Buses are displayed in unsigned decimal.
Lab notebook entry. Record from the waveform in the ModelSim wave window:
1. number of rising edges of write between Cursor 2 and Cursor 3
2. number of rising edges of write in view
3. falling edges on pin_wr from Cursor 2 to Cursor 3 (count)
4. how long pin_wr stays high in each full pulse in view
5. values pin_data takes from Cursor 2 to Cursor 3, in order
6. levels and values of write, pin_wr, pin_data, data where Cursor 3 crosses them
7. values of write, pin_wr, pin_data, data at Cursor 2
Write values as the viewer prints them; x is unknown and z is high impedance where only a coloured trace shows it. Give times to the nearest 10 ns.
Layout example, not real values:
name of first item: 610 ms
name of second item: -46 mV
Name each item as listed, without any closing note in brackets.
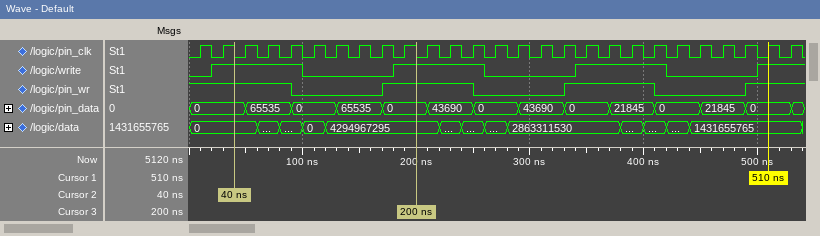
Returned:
number of rising edges of write between Cursor 2 and Cursor 3: 1
number of rising edges of write in view: 4
falling edges on pin_wr from Cursor 2 to Cursor 3: 1
how long pin_wr stays high in each full pulse in view: 80 ns, 80 ns
values pin_data takes from Cursor 2 to Cursor 3, in order: 0, 65535, 0, 65535, 0
levels and values of write, pin_wr, pin_data, data where Cursor 3 crosses them: write=1, pin_wr=1, pin_data=0, data=4294967295
values of write, pin_wr, pin_data, data at Cursor 2: write=1, pin_wr=1, pin_data=0, data=0
